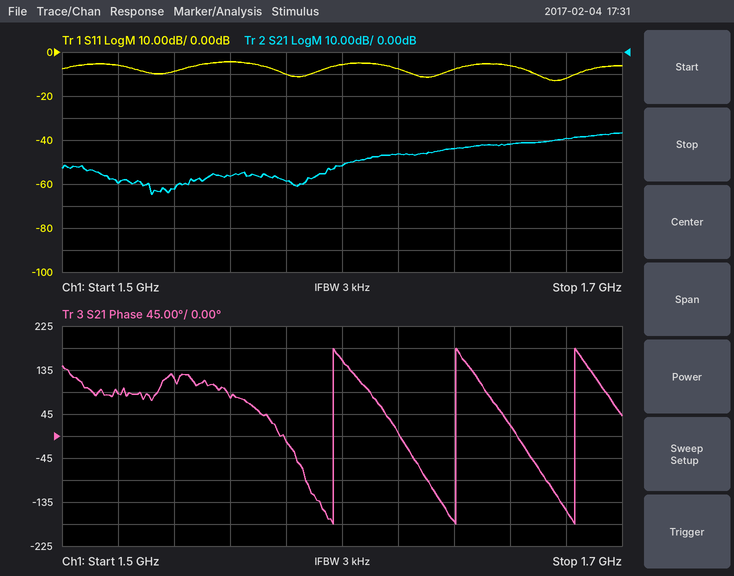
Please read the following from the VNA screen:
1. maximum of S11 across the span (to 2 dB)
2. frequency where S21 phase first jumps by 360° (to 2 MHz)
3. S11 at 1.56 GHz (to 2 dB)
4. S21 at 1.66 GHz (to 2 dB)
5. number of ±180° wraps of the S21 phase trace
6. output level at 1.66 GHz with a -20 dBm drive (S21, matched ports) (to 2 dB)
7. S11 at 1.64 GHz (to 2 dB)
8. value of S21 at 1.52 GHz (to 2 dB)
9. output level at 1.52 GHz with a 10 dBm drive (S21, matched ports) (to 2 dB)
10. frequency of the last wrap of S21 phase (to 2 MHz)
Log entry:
-4 dB
1.596 GHz
-4 dB
-42 dB
3
-62 dBm
-8 dB
-60 dB
-50 dBm
1.684 GHz
